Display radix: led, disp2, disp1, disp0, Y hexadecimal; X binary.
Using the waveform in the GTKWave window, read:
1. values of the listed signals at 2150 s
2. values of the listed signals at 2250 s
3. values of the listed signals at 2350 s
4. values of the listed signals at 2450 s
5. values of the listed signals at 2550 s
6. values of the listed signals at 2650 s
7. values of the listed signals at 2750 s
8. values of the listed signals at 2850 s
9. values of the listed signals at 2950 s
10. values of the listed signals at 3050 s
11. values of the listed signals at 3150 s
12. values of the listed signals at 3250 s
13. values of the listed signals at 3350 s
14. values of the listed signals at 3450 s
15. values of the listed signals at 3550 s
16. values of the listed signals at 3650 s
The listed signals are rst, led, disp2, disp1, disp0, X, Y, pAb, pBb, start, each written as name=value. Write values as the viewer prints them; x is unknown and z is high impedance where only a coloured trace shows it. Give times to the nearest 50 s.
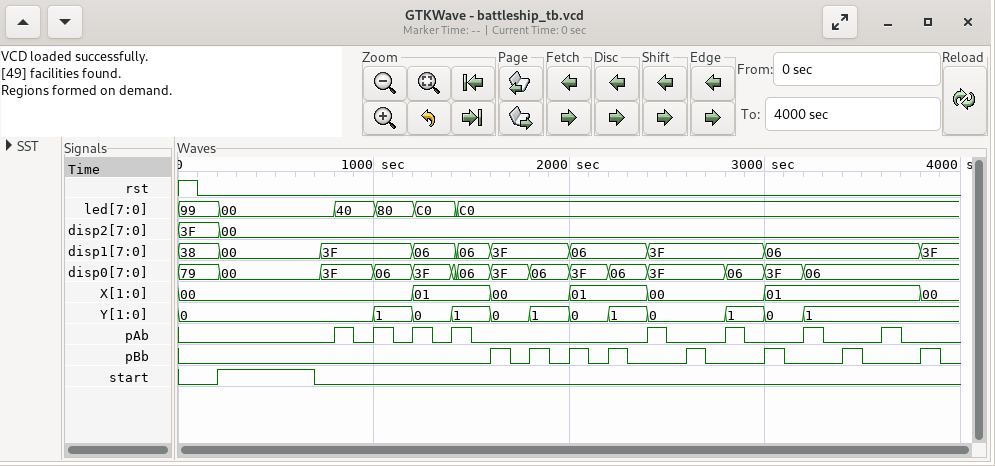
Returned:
rst=0, led=C0, disp2=00, disp1=06, disp0=3F, X=01, Y=0, pAb=0, pBb=0, start=0
rst=0, led=C0, disp2=00, disp1=06, disp0=06, X=01, Y=1, pAb=0, pBb=1, start=0
rst=0, led=C0, disp2=00, disp1=06, disp0=06, X=01, Y=1, pAb=0, pBb=0, start=0
rst=0, led=C0, disp2=00, disp1=3F, disp0=3F, X=00, Y=0, pAb=1, pBb=0, start=0
rst=0, led=C0, disp2=00, disp1=3F, disp0=3F, X=00, Y=0, pAb=0, pBb=0, start=0
rst=0, led=C0, disp2=00, disp1=3F, disp0=3F, X=00, Y=0, pAb=0, pBb=1, start=0
rst=0, led=C0, disp2=00, disp1=3F, disp0=3F, X=00, Y=0, pAb=0, pBb=0, start=0
rst=0, led=C0, disp2=00, disp1=3F, disp0=06, X=00, Y=1, pAb=1, pBb=0, start=0
rst=0, led=C0, disp2=00, disp1=3F, disp0=06, X=00, Y=1, pAb=0, pBb=0, start=0
rst=0, led=C0, disp2=00, disp1=06, disp0=3F, X=01, Y=0, pAb=0, pBb=1, start=0
rst=0, led=C0, disp2=00, disp1=06, disp0=3F, X=01, Y=0, pAb=0, pBb=0, start=0
rst=0, led=C0, disp2=00, disp1=06, disp0=06, X=01, Y=1, pAb=1, pBb=0, start=0
rst=0, led=C0, disp2=00, disp1=06, disp0=06, X=01, Y=1, pAb=0, pBb=0, start=0
rst=0, led=C0, disp2=00, disp1=06, disp0=06, X=01, Y=1, pAb=0, pBb=1, start=0
rst=0, led=C0, disp2=00, disp1=06, disp0=06, X=01, Y=1, pAb=0, pBb=0, start=0
rst=0, led=C0, disp2=00, disp1=06, disp0=06, X=01, Y=1, pAb=1, pBb=0, start=0
